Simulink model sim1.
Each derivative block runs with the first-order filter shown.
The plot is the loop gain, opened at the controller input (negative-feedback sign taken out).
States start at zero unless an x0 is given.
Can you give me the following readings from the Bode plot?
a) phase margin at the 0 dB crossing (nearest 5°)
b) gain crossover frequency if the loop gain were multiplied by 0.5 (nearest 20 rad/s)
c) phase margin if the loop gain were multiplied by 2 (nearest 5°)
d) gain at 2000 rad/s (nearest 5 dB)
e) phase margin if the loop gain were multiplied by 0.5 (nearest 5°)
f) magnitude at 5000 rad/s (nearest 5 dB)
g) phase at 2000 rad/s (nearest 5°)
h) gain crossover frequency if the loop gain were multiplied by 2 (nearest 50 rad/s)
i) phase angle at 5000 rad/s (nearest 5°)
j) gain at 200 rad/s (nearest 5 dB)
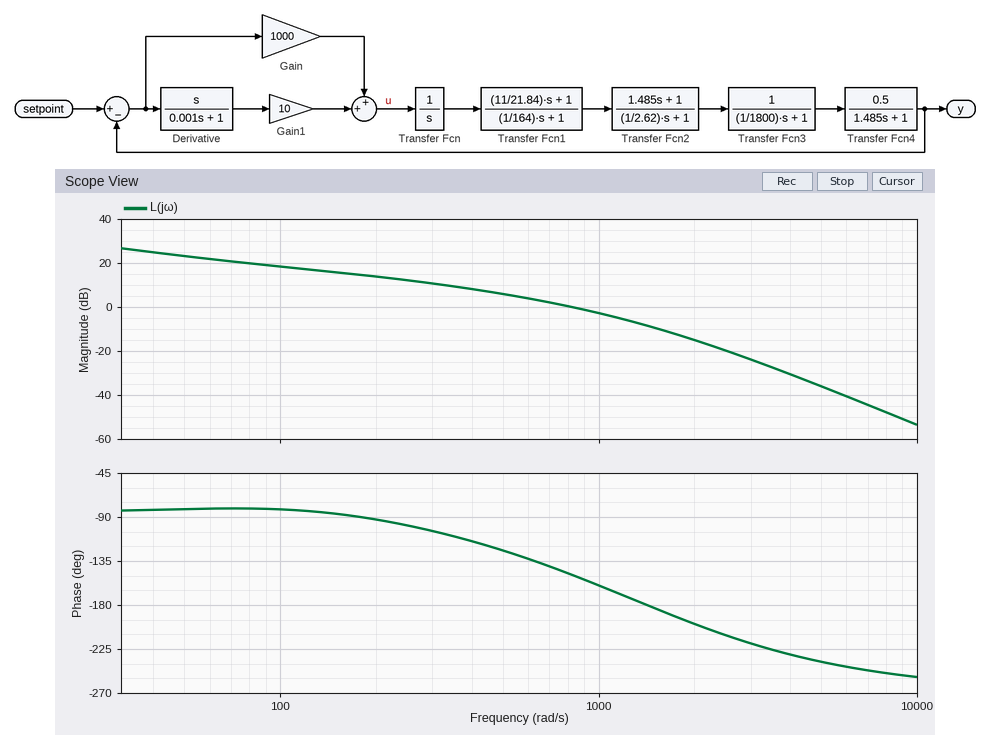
30°
500 rad/s
10°
-15 dB
55°
-35 dB
-200°
1250 rad/s
-240°
15 dB
